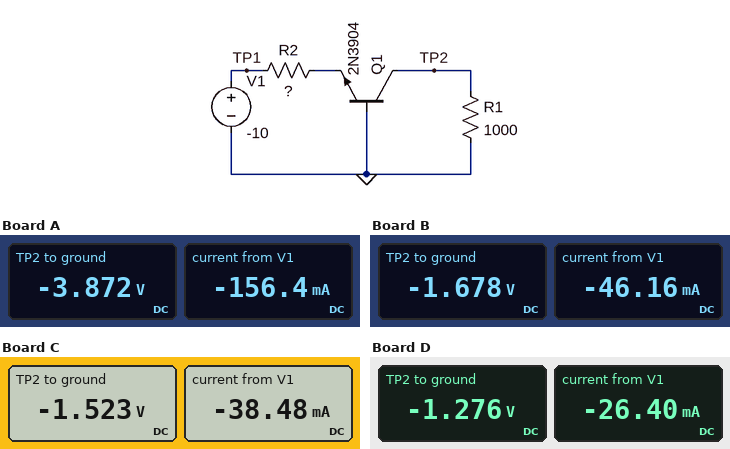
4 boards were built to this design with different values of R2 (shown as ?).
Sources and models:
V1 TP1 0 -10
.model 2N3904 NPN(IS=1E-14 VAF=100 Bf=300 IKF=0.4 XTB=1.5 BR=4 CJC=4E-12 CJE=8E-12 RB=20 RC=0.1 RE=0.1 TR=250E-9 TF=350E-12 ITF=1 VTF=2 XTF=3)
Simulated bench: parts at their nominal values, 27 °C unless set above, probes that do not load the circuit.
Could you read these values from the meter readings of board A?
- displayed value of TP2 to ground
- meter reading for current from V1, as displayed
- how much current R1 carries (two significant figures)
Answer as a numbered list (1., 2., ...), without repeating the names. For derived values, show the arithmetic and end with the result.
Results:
1. -3.872 V
2. -156.4 mA
3. (0 V - (-3.872 V)) / 1 kΩ = 3.9 mA
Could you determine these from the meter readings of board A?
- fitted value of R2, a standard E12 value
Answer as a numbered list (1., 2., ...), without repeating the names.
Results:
1. 39 Ω
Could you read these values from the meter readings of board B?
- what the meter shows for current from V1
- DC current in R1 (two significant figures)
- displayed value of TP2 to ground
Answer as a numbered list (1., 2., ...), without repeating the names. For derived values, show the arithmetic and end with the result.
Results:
1. -46.16 mA
2. (0 V - (-1.678 V)) / 1 kΩ = 1.7 mA
3. -1.678 V
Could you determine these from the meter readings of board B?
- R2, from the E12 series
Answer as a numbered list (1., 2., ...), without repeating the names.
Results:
1. 180 Ω
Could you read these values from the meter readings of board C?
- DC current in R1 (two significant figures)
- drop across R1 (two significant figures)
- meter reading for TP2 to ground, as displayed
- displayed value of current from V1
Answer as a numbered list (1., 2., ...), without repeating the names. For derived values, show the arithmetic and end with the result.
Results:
1. (0 V - (-1.523 V)) / 1 kΩ = 1.5 mA
2. 0 V - (-1.523 V) = 1.5 V
3. -1.523 V
4. -38.48 mA
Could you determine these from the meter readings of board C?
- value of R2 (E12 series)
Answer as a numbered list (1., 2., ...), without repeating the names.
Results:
1. 220 Ω
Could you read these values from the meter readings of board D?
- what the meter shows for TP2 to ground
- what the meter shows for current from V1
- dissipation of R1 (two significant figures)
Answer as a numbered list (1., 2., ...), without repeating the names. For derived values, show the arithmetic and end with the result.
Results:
1. -1.276 V
2. -26.40 mA
3. (0 V - (-1.276 V))^2 / 1 kΩ = 1.6 mW
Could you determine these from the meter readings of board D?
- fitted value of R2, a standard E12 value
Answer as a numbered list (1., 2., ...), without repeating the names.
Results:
1. 330 Ω
